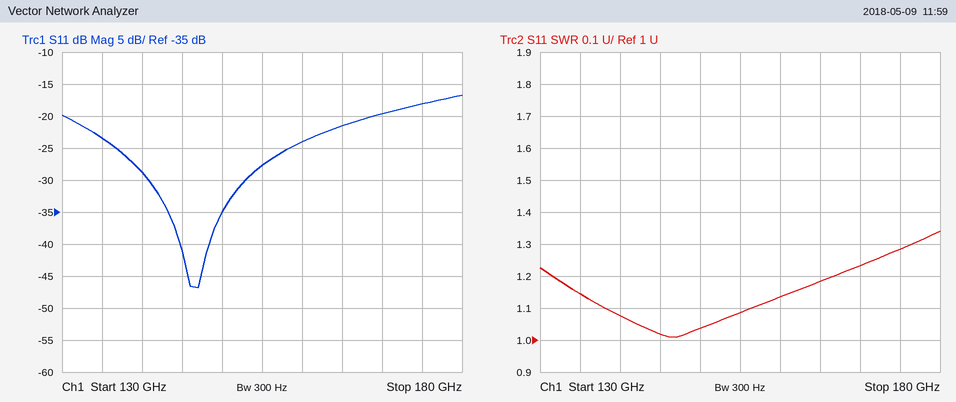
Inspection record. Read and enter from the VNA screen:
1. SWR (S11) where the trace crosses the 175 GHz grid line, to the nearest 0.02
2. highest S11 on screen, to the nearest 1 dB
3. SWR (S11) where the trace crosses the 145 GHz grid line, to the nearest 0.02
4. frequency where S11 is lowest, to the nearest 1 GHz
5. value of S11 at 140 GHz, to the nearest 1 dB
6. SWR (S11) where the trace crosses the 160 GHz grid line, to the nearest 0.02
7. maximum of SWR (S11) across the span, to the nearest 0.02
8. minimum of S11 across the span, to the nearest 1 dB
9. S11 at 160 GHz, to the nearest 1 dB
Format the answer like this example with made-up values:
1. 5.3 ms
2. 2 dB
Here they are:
1. 1.28
2. -17 dB
3. 1.02
4. 147 GHz
5. -29 dB
6. 1.14
7. 1.34
8. -47 dB
9. -24 dB
